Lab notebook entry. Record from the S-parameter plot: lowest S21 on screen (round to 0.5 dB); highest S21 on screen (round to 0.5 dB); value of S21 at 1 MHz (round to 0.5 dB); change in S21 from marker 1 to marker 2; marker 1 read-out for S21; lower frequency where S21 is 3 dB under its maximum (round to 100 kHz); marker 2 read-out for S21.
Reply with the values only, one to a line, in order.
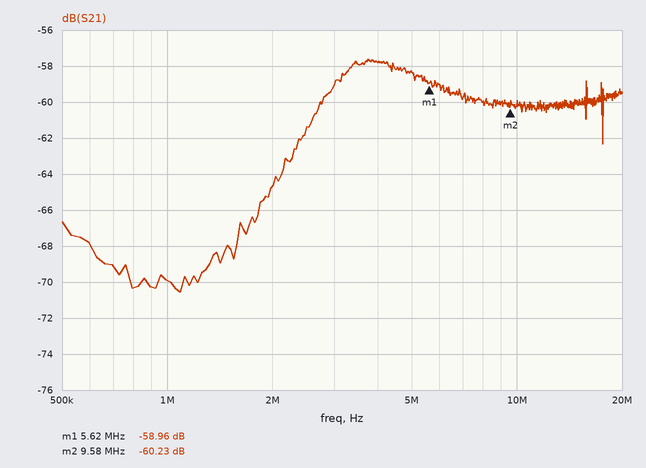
-70.5 dB
-57.5 dB
-70.0 dB
-1.27 dB
-58.96 dB
2.7 MHz
-60.23 dB
